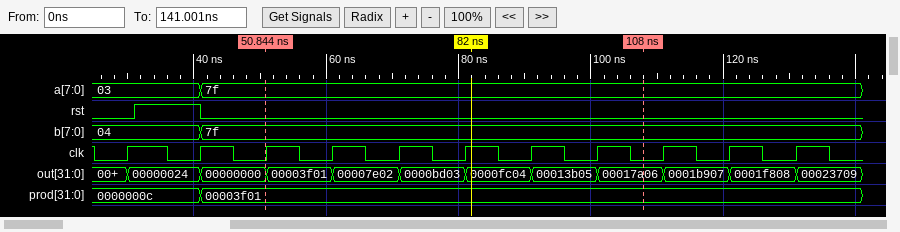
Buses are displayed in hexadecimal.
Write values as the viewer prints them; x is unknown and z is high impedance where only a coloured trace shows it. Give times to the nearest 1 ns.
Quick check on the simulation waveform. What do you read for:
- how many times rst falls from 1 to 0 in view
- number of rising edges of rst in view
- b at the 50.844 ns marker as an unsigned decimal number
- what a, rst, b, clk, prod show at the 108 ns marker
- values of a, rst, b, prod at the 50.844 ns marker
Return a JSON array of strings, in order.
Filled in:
["1", "1", "127", "a=7f, rst=0, b=7f, clk=0, prod=00003f01", "a=7f, rst=0, b=7f, prod=00003f01"]
